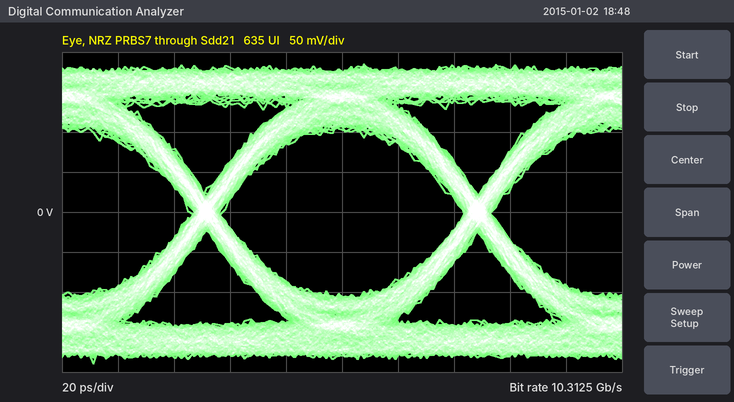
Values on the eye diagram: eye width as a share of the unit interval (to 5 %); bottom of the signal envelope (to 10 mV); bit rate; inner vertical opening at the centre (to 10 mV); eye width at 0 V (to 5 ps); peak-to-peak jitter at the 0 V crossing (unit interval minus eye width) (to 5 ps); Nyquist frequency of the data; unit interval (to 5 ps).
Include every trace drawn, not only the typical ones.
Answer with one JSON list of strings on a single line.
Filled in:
["90 %", "-190 mV", "10.3125 Gb/s", "210 mV", "85 ps", "10 ps", "5.15625 GHz", "95 ps"]
